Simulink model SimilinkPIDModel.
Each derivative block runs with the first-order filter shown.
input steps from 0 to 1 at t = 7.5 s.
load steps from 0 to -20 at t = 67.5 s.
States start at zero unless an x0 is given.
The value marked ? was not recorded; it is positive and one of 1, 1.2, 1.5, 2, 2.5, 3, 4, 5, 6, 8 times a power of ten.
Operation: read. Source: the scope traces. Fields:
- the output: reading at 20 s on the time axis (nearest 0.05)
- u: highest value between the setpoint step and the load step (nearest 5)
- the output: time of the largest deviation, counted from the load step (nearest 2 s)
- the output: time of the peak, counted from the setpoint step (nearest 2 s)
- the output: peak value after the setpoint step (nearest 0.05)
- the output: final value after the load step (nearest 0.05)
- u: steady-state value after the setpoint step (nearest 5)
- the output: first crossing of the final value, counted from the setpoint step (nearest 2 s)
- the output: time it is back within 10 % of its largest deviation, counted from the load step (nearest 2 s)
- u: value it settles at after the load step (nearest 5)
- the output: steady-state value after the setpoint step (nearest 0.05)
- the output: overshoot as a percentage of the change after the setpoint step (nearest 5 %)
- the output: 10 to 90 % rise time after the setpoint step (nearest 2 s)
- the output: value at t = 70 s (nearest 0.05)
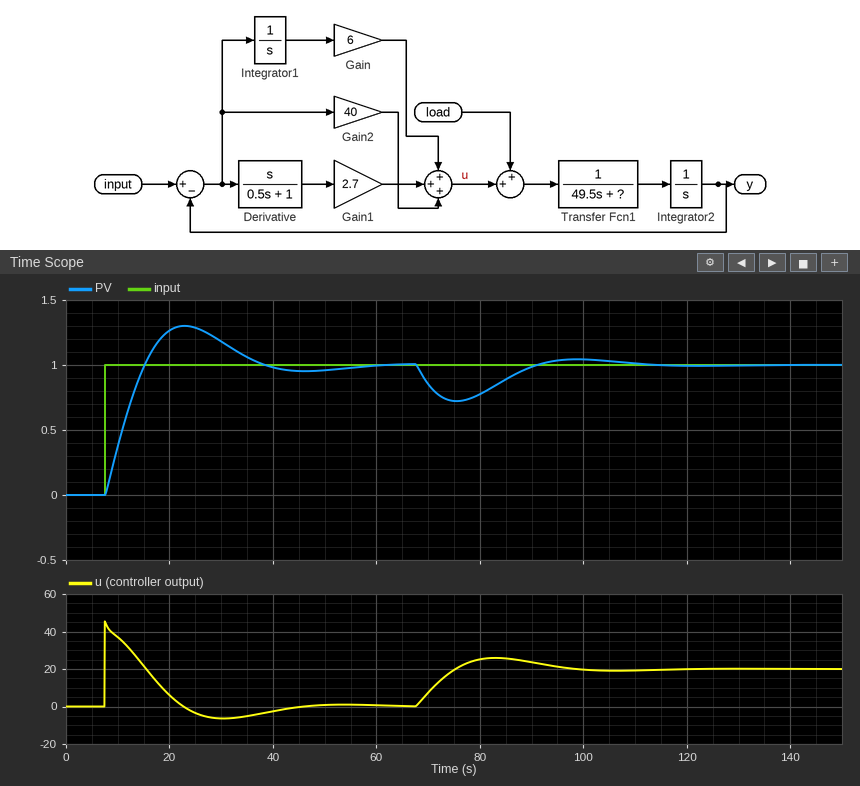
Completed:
1.25
45
8 s
16 s
1.30
1.00
0
8 s
38 s
20
1.00
30 %
6 s
0.85
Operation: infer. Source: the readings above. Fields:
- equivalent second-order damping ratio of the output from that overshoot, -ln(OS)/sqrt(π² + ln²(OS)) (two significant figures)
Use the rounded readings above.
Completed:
0.36
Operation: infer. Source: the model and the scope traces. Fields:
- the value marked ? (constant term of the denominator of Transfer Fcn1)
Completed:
250
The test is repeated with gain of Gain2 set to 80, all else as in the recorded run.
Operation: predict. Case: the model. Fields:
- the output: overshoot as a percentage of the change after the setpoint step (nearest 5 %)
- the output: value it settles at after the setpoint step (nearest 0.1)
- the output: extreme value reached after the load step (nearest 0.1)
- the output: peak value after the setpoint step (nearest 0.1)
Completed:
15 %
1.0
0.8
1.1
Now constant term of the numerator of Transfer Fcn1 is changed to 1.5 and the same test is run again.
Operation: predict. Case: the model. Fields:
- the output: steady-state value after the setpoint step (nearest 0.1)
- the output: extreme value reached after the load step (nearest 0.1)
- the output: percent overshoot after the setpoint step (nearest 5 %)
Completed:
1.0
0.7
25 %
